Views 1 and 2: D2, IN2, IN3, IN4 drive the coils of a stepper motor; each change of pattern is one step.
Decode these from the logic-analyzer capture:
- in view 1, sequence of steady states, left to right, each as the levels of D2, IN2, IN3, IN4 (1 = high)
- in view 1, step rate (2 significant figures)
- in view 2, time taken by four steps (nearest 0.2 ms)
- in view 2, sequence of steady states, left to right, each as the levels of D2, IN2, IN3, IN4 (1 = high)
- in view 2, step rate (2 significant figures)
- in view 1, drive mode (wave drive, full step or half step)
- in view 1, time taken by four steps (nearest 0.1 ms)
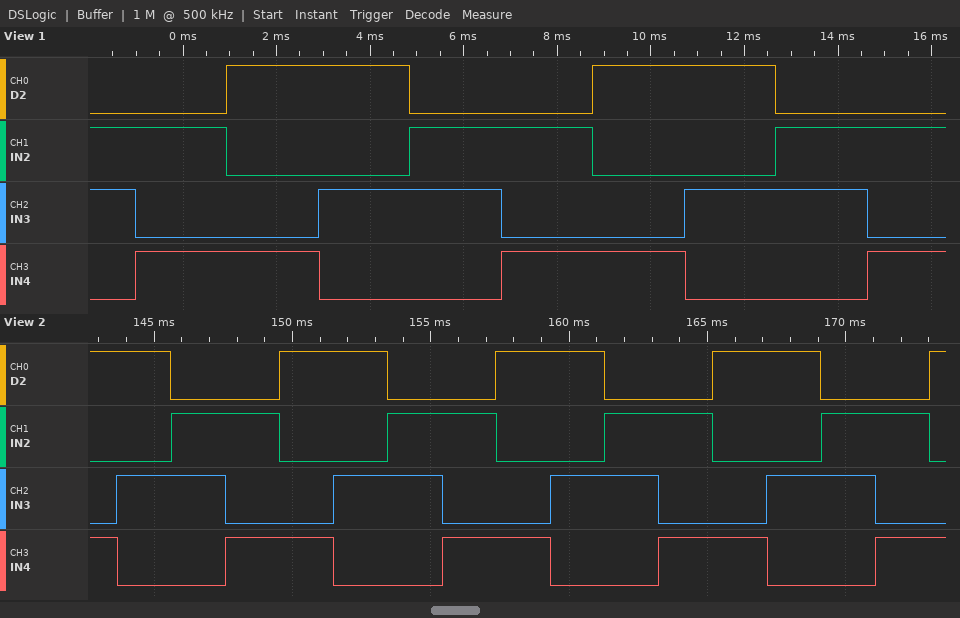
0110 0101 1001 1010 0110 0101 1001 1010 0110 0101
510 steps/s
7.8 ms
1001 1010 0110 0101 1001 1010 0110 0101 1001 1010 0110 0101 1001 1010 0110 0101 1001
510 steps/s
full step
7.8 ms
